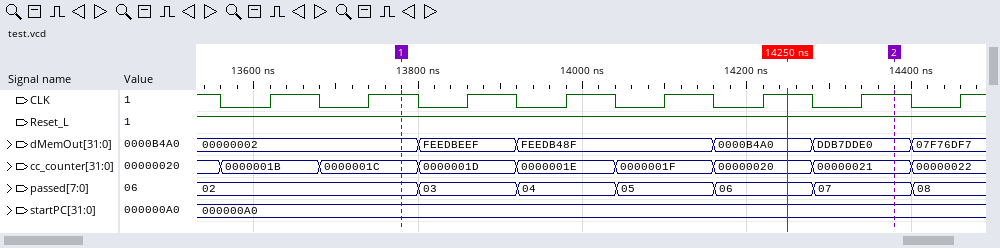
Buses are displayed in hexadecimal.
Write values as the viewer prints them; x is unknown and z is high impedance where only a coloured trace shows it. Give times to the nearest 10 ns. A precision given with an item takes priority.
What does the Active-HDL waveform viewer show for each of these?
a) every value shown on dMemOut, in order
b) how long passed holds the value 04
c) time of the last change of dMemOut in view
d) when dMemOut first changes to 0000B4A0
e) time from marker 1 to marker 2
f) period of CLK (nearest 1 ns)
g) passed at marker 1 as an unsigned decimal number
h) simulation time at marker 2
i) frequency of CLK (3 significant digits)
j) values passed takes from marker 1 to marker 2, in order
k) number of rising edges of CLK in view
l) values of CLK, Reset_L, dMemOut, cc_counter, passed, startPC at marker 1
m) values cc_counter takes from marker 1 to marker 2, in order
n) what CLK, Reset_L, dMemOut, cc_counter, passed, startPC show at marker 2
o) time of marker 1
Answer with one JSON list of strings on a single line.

["00000002, FEEDBEEF, FEEDB48F, 0000B4A0, DDB7DDE0, 07F76DF7", "120 ns", "14400 ns", "14160 ns", "600 ns", "120 ns", "2", "14380 ns", "8.33 MHz", "02, 03, 04, 05, 06, 07", "8", "CLK=1, Reset_L=1, dMemOut=00000002, cc_counter=0000001C, passed=02, startPC=000000A0", "0000001C, 0000001D, 0000001E, 0000001F, 00000020, 00000021", "CLK=1, Reset_L=1, dMemOut=DDB7DDE0, cc_counter=00000021, passed=07, startPC=000000A0", "13780 ns"]
